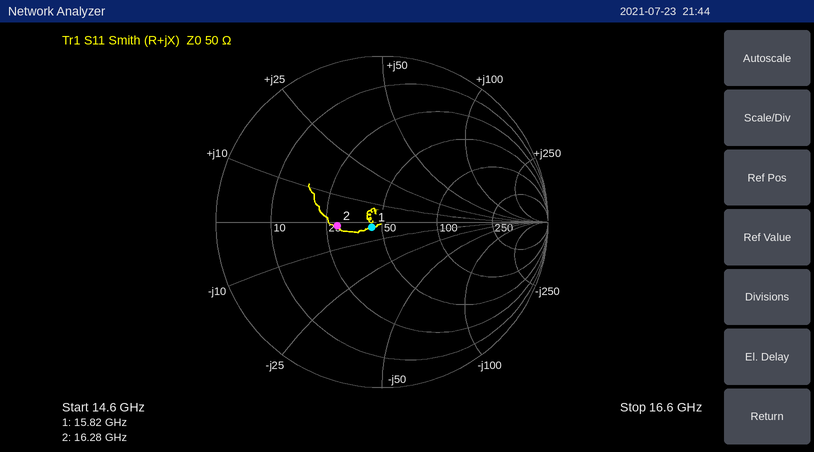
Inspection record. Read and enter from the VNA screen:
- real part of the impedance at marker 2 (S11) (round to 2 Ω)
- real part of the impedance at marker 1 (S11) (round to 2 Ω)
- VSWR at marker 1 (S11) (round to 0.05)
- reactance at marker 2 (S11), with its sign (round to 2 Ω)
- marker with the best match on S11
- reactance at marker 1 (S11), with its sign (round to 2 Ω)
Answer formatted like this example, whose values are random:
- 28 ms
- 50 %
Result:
- 28 Ω
- 44 Ω
- 1.15
- -2 Ω
- marker 1
- -2 Ω
